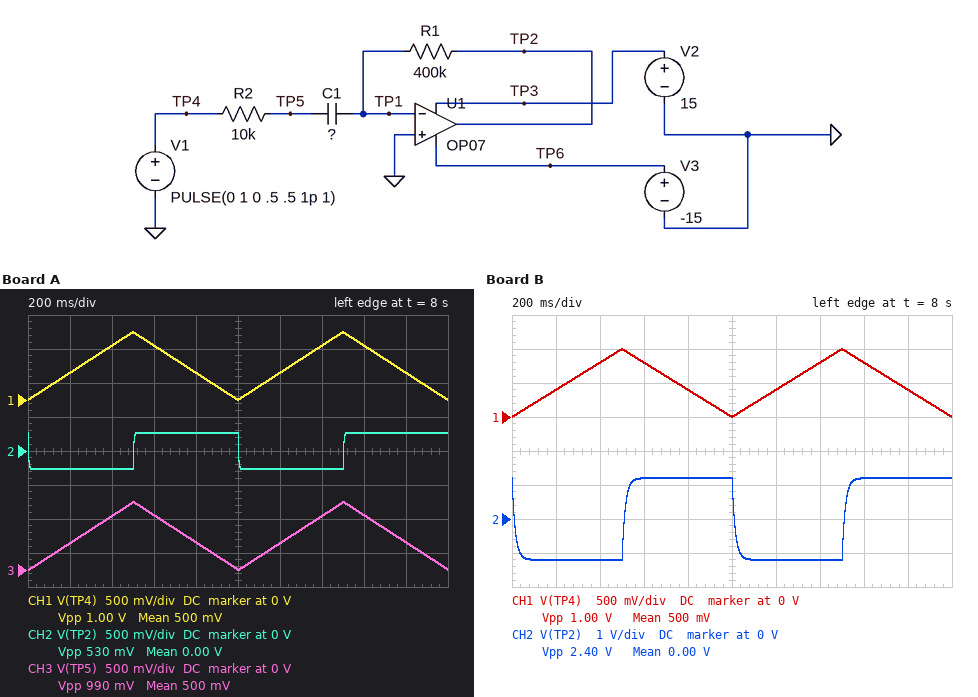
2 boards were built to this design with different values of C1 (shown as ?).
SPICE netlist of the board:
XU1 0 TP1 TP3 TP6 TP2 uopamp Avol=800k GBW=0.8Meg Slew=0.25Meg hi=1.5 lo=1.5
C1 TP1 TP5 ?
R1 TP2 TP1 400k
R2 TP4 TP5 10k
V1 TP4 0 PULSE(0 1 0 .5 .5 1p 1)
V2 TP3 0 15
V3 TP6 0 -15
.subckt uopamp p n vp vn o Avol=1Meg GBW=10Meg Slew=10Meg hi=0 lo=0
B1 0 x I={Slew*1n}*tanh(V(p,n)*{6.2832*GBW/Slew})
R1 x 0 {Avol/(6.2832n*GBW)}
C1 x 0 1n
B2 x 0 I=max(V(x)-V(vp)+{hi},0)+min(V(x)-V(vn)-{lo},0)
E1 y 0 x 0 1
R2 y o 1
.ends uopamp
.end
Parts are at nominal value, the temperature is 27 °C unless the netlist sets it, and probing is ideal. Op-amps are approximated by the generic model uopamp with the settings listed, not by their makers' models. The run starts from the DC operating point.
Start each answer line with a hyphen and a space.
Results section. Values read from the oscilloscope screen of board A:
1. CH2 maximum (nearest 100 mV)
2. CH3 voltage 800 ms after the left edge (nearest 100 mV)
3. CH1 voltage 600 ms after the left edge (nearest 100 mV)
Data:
- 300 mV
- 400 mV
- 800 mV
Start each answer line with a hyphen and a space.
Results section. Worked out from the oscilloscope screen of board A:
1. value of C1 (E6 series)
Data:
- 330 nF
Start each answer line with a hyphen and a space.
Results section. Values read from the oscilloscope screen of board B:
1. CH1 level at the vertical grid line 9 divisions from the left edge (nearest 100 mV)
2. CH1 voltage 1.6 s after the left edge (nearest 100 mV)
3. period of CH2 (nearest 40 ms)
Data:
- 400 mV
- 800 mV
- 1.00 s
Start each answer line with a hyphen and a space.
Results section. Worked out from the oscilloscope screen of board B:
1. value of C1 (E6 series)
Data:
- 1.5 µF
